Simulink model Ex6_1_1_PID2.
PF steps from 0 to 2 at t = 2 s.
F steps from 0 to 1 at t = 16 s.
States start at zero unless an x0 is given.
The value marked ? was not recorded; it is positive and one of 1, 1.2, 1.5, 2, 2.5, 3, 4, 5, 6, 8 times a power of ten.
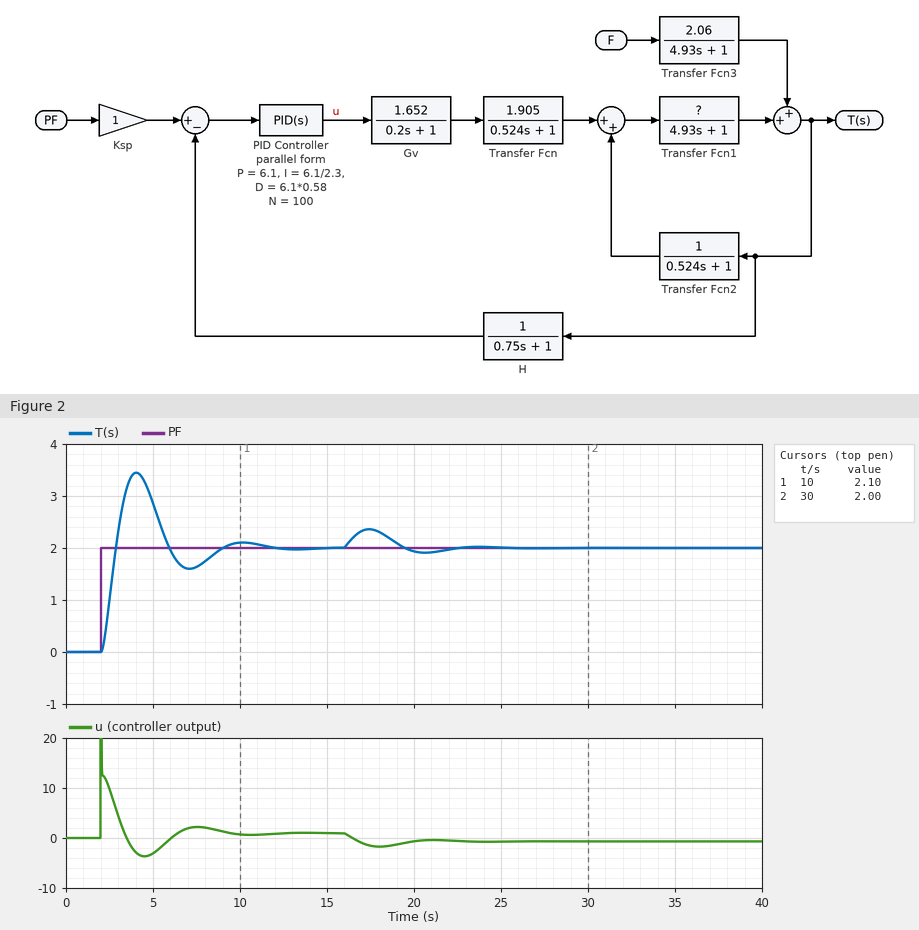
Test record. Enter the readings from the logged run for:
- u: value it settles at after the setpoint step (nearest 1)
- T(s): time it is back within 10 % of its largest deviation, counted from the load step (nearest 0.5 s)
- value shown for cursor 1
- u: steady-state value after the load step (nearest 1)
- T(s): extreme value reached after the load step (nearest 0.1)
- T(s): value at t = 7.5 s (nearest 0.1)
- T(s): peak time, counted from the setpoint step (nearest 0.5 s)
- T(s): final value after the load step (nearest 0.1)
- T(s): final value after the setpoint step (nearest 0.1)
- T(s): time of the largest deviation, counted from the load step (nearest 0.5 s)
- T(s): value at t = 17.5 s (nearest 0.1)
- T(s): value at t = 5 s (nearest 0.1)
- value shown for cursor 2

1
6.0 s
2.10
-1
2.4
1.6
2.0 s
2.0
2.0
1.5 s
2.4
2.9
2.00
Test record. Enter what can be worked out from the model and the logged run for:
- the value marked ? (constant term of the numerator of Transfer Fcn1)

0.4
